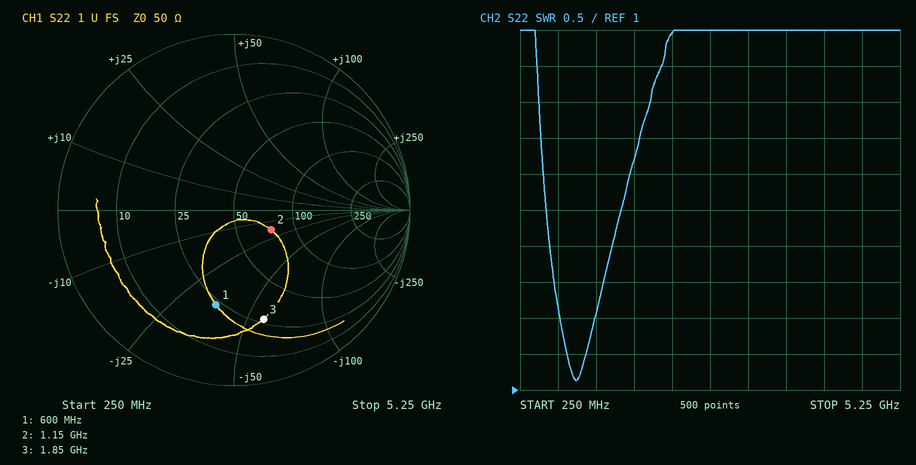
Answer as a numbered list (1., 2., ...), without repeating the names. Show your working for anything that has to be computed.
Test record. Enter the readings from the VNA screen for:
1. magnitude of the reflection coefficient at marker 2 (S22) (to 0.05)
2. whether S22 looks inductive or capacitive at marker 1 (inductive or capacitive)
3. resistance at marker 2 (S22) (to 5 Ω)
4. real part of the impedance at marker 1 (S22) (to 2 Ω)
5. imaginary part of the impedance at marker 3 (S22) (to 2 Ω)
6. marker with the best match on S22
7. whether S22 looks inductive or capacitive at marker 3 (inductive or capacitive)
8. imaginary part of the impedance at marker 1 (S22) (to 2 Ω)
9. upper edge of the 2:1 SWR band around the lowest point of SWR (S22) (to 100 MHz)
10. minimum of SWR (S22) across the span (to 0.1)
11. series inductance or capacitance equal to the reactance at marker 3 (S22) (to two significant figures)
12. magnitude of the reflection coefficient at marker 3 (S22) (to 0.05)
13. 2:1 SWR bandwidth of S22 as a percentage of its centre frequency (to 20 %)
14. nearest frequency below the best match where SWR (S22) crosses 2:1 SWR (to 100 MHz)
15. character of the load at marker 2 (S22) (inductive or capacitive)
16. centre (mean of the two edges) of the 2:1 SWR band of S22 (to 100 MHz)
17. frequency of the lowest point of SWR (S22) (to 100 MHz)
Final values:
1. 0.25
2. capacitive
3. 75 Ω
4. 24 Ω
5. -58 Ω
6. marker 2
7. capacitive
8. -36 Ω
9. 1.2 GHz
10. 1.1
11. C = 1/(2π × 1.85 GHz × 58 Ω) ≈ 1.5 pF
12. 0.65
13. 400 MHz / 1 GHz ≈ 40 %
14. 800 MHz
15. capacitive
16. 1.0 GHz
17. 1.0 GHz
